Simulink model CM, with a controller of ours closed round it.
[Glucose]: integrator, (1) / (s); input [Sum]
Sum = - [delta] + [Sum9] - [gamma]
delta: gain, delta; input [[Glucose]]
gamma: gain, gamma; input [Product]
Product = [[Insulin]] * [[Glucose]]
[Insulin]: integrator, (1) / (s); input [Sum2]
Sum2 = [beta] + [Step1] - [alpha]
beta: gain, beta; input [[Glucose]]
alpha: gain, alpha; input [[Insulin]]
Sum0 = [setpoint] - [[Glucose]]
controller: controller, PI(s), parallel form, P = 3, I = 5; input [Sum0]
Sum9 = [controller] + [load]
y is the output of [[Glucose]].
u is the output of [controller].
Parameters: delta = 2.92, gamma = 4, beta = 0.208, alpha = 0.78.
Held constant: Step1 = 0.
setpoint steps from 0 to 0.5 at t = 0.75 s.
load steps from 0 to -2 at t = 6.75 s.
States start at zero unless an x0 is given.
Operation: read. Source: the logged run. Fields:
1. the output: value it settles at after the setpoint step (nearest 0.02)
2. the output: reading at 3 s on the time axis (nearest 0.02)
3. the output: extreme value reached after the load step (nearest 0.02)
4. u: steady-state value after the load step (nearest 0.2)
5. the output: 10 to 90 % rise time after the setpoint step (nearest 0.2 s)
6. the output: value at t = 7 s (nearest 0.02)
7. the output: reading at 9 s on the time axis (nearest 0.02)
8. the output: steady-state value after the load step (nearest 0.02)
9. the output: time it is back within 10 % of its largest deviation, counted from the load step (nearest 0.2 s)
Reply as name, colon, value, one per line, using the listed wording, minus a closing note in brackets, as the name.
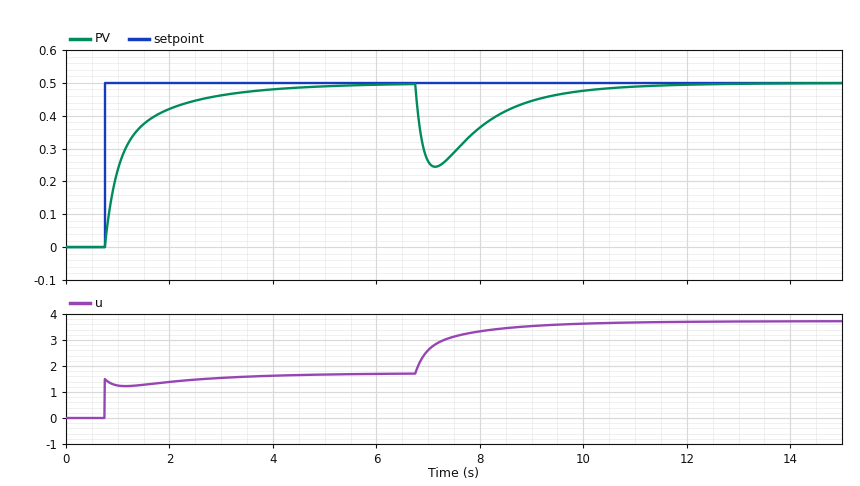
the output: value it settles at after the setpoint step: 0.50
the output: reading at 3 s on the time axis: 0.46
the output: extreme value reached after the load step: 0.24
u: steady-state value after the load step: 3.8
the output: 10 to 90 % rise time after the setpoint step: 1.8 s
the output: value at t = 7 s: 0.26
the output: reading at 9 s on the time axis: 0.44
the output: steady-state value after the load step: 0.50
the output: time it is back within 10 % of its largest deviation, counted from the load step: 3.2 s
